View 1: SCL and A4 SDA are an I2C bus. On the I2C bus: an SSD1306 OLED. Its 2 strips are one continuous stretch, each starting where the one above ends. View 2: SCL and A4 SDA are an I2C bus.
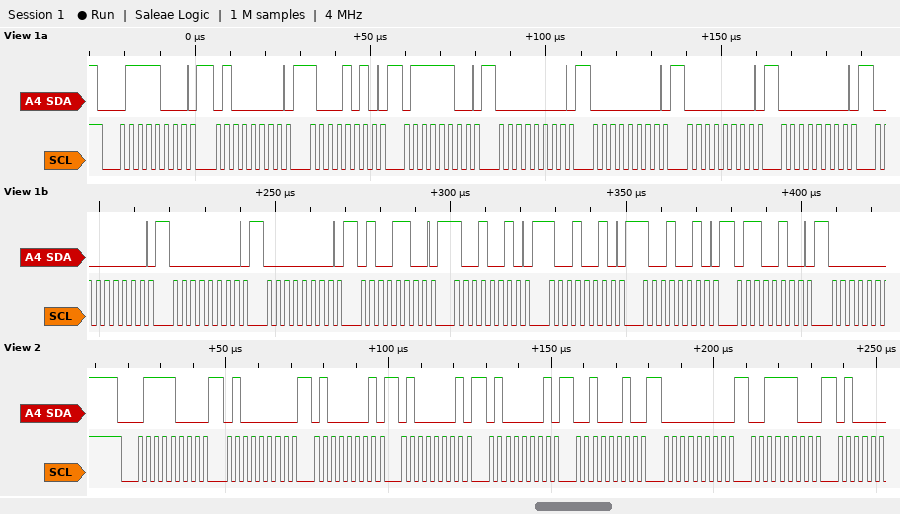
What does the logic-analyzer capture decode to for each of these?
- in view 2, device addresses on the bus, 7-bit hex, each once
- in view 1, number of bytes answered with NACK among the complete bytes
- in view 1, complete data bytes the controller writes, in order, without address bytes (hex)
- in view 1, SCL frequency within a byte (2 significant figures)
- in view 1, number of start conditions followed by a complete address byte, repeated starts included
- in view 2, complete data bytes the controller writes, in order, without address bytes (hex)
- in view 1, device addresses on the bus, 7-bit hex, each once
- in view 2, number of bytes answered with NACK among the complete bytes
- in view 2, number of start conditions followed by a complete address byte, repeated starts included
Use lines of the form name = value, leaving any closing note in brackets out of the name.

in view 2, device addresses on the bus, 7-bit hex, each once = 0x3C
in view 1, number of bytes answered with NACK among the complete bytes = 0
in view 1, complete data bytes the controller writes, in order, without address bytes = 40 8A 7C 00 00 00 00 00 00 00 4C 92 92 92 64
in view 1, SCL frequency within a byte = 400 kHz
in view 1, number of start conditions followed by a complete address byte, repeated starts included = 1
in view 2, complete data bytes the controller writes, in order, without address bytes = 40 41 41 41 22 00 3C
in view 1, device addresses on the bus, 7-bit hex, each once = 0x3C
in view 2, number of bytes answered with NACK among the complete bytes = 0
in view 2, number of start conditions followed by a complete address byte, repeated starts included = 1
